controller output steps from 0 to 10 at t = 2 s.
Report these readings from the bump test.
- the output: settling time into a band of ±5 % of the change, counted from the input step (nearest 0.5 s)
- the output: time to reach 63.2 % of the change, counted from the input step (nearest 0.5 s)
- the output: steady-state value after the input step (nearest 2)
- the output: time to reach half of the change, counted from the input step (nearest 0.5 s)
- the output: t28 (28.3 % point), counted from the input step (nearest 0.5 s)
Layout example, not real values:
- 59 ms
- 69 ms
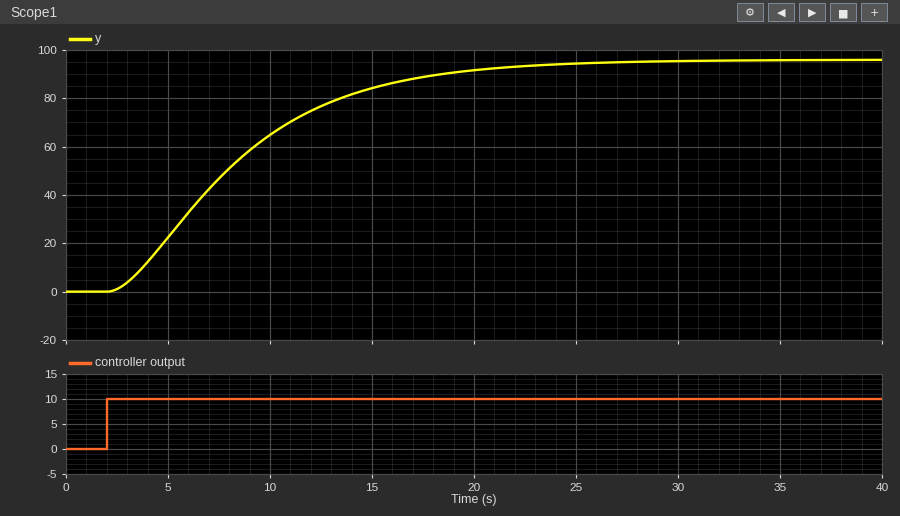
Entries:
- 17.5 s
- 7.5 s
- 96
- 5.5 s
- 3.5 s
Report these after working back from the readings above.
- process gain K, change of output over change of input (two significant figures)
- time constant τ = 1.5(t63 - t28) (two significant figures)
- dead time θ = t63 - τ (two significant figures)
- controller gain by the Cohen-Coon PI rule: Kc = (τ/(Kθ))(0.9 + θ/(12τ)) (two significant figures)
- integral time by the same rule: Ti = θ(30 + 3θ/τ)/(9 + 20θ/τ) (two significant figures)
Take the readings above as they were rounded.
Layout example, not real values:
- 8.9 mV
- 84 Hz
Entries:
- 9.6
- 6.0 s
- 1.5 s
- 0.38
- 3.3 s
